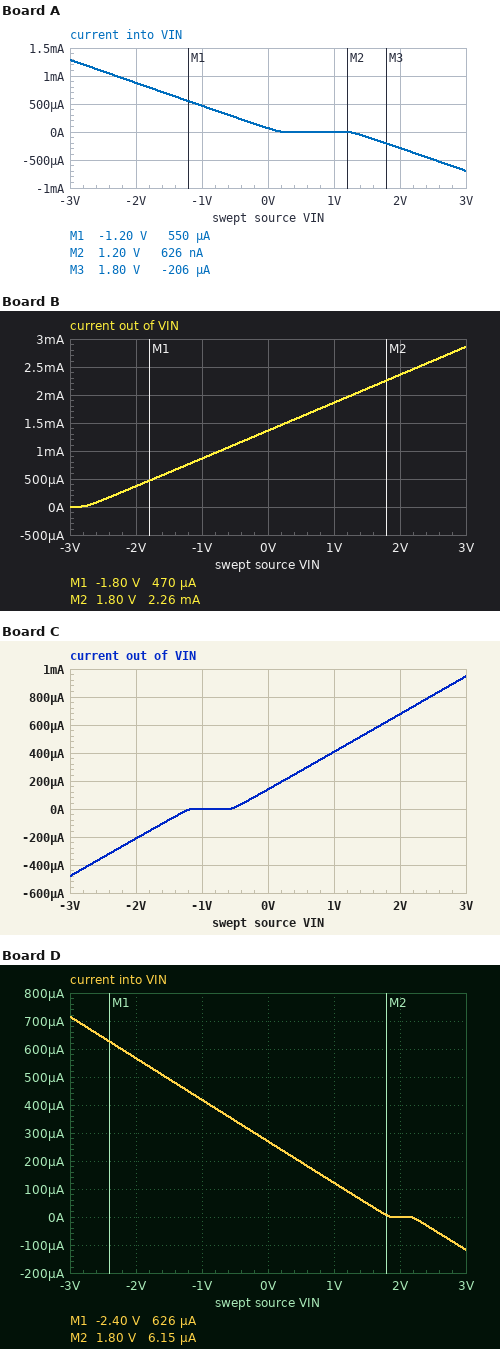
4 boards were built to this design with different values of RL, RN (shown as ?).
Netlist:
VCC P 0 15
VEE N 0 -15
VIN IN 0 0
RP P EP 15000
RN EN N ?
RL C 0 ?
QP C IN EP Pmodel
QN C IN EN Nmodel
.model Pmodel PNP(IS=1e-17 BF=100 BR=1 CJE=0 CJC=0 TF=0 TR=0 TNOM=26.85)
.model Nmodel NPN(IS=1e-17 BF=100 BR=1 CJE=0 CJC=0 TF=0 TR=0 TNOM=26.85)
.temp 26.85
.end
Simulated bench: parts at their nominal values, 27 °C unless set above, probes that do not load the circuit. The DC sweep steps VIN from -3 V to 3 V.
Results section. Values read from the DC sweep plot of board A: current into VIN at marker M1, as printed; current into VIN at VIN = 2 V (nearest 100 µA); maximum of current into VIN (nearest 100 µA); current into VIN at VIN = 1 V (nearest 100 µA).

550 µA
-300 µA
1.3 mA
0 A
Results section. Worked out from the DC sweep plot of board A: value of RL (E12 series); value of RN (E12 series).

3.3 kΩ
22 kΩ
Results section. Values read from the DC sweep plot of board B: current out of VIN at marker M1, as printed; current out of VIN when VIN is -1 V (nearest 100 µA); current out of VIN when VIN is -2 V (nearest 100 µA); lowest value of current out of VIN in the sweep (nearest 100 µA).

470 µA
900 µA
400 µA
0 A
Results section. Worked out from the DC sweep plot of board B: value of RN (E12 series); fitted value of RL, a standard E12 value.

5.6 kΩ
3.9 kΩ
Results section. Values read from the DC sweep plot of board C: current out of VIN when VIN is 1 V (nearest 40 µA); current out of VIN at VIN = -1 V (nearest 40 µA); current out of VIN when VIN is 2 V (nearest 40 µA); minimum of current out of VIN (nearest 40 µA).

400 µA
0 A
680 µA
-480 µA
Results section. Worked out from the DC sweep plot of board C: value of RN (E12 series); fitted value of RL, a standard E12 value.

12 kΩ
8.2 kΩ
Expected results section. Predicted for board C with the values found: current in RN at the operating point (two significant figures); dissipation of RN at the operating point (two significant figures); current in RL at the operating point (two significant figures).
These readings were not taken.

1.2 mA
17 mW
95 µA
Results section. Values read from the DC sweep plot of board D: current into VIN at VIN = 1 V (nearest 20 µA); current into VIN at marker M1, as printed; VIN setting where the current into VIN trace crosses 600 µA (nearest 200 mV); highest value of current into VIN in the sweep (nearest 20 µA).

120 µA
626 µA
-2.2 V
720 µA
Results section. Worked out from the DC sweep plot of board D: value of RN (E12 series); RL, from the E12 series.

22 kΩ
27 kΩ
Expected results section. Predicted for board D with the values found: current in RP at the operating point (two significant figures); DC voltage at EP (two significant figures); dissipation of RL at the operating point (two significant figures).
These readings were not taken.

940 µA
840 mV
24 µW
